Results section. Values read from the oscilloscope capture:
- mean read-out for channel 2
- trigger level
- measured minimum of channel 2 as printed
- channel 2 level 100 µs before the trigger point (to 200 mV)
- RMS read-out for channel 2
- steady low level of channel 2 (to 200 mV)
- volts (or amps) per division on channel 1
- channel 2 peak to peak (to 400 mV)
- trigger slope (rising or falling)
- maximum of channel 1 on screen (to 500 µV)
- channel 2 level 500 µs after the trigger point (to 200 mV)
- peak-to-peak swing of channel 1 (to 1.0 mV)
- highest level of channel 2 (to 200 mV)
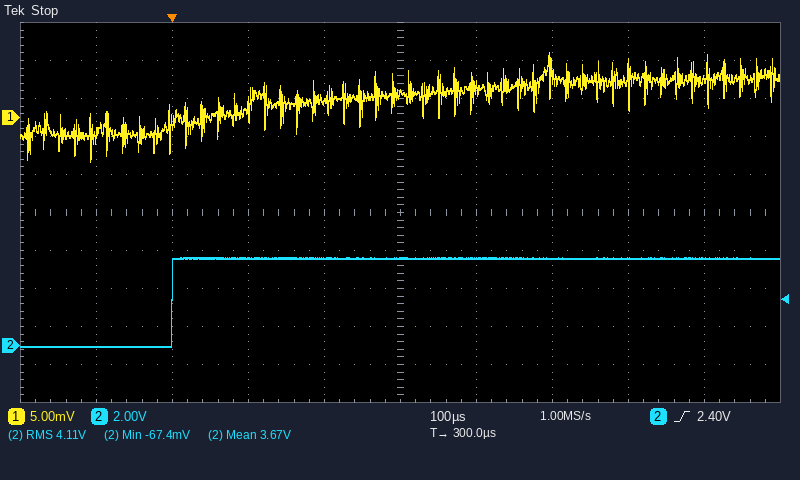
3.67 V
2.40 V
-67.4 mV
0.0 V
4.11 V
0.0 V
5 mV
4.8 V
rising
8.5 mV
4.6 V
14.0 mV
4.6 V
